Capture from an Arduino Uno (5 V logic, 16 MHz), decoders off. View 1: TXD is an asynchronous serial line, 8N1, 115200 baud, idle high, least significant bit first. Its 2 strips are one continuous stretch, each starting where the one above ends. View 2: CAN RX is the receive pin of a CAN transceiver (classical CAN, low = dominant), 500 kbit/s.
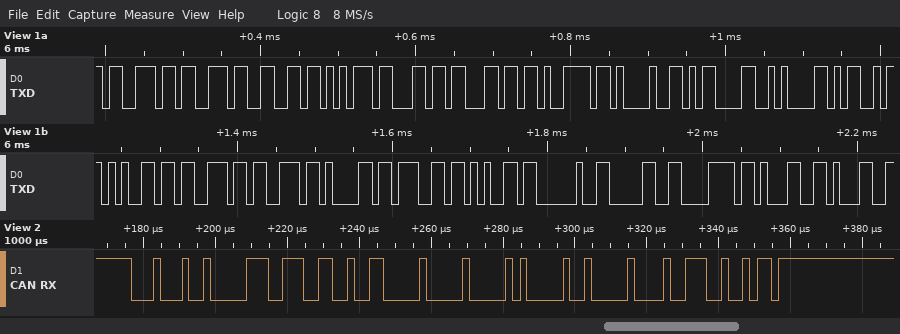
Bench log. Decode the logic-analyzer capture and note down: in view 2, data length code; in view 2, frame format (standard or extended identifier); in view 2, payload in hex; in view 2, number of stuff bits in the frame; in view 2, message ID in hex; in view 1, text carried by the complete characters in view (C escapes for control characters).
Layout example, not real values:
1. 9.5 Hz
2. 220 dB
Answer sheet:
1. 6
2. standard
3. 73 26 00 01 01 00
4. 6
5. 0x112
6. "ssfully!\r\nMessage 0x11"
